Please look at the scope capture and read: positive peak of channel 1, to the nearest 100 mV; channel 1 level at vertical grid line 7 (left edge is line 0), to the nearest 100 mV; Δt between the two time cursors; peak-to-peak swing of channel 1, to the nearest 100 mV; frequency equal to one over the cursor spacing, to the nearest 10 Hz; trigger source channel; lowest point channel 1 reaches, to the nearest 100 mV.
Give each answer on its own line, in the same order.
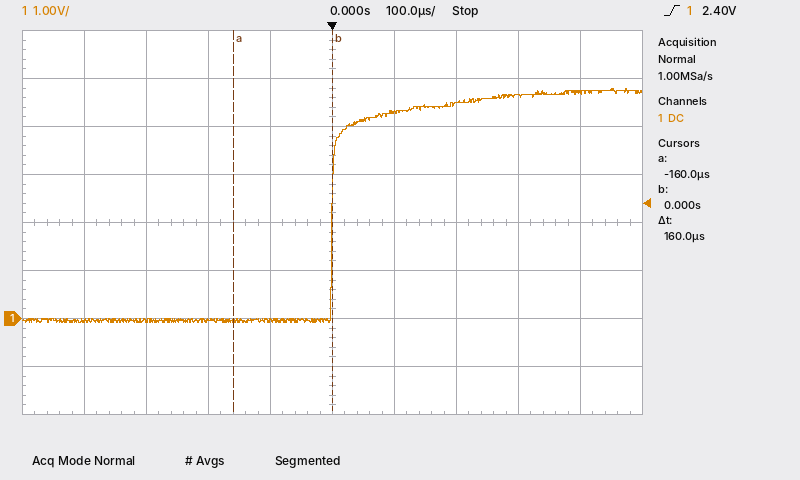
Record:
4.8 V
4.5 V
160 µs
4.9 V
6.25 kHz
channel 1
-100 mV
